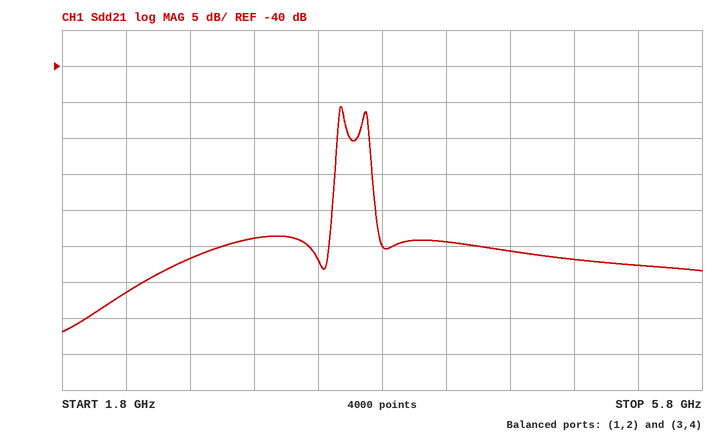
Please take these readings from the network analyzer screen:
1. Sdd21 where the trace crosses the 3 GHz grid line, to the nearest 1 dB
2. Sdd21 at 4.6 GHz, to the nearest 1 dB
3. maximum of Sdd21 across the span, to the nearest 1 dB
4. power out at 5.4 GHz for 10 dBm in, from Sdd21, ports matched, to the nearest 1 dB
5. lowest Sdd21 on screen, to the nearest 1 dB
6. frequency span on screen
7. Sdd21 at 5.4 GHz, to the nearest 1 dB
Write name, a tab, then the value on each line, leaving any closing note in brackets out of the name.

Sdd21 where the trace crosses the 3 GHz grid line, to the nearest 1 dB	-64 dB
Sdd21 at 4.6 GHz, to the nearest 1 dB	-66 dB
maximum of Sdd21 across the span, to the nearest 1 dB	-46 dB
power out at 5.4 GHz for 10 dBm in, from Sdd21, ports matched, to the nearest 1 dB	-58 dBm
lowest Sdd21 on screen, to the nearest 1 dB	-77 dB
frequency span on screen	4 GHz
Sdd21 at 5.4 GHz, to the nearest 1 dB	-68 dB
